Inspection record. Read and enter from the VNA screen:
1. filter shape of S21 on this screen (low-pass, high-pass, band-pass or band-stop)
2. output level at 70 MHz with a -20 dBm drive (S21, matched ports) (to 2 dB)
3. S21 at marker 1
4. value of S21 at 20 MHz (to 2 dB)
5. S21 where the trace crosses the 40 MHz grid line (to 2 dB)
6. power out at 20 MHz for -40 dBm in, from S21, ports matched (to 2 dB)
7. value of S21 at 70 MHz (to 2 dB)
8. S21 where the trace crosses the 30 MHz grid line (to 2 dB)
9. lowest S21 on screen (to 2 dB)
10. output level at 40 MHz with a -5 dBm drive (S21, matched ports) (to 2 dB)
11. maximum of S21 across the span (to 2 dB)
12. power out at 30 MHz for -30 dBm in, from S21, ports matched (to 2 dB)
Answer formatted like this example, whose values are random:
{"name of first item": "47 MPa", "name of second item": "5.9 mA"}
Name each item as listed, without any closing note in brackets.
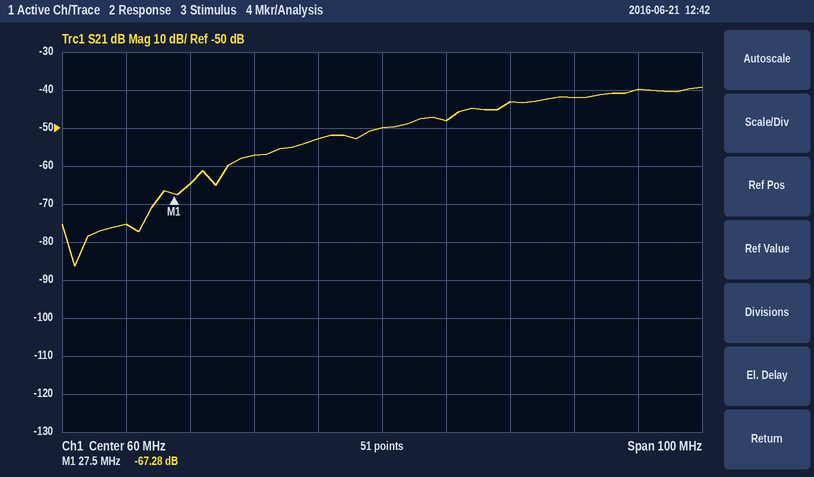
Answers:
{"filter shape of S21 on this screen": "high-pass", "output level at 70 MHz with a -20 dBm drive (S21, matched ports)": "-68 dBm", "S21 at marker 1": "-67.28 dB", "value of S21 at 20 MHz": "-76 dB", "S21 where the trace crosses the 40 MHz grid line": "-58 dB", "power out at 20 MHz for -40 dBm in, from S21, ports matched": "-116 dBm", "value of S21 at 70 MHz": "-48 dB", "S21 where the trace crosses the 30 MHz grid line": "-64 dB", "lowest S21 on screen": "-86 dB", "output level at 40 MHz with a -5 dBm drive (S21, matched ports)": "-62 dBm", "maximum of S21 across the span": "-40 dB", "power out at 30 MHz for -30 dBm in, from S21, ports matched": "-94 dBm"}
